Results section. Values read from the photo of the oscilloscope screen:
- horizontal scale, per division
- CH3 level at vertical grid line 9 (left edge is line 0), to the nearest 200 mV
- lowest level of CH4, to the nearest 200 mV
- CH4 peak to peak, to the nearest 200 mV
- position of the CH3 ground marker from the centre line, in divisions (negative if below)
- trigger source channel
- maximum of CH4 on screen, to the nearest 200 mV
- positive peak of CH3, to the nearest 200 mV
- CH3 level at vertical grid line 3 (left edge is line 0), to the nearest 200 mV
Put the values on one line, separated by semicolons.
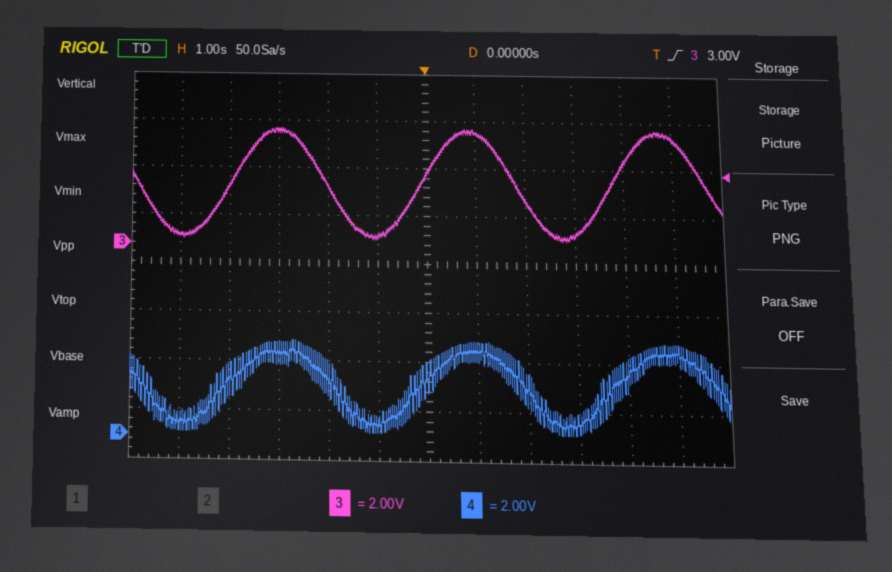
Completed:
1 s; 400 mV; 200 mV; 3.6 V; +0.4 div; CH3; 3.8 V; 4.8 V; 4.8 V
